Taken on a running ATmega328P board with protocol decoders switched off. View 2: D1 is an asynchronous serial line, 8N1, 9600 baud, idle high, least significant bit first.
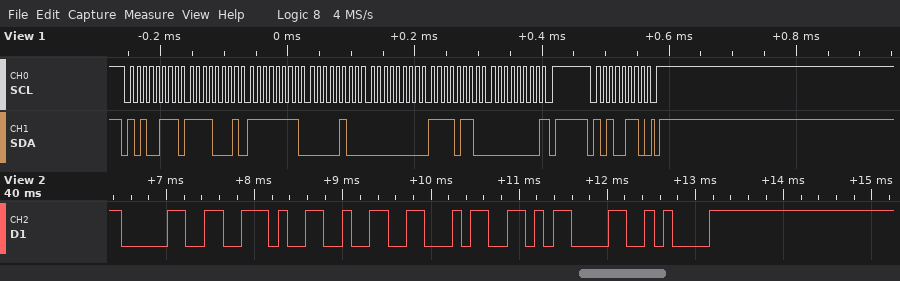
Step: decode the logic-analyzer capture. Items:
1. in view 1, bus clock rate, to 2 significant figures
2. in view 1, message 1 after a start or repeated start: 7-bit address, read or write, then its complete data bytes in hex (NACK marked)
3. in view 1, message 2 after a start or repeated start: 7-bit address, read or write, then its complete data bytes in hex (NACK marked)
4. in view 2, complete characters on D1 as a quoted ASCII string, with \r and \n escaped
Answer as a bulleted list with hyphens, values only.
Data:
- 100 kHz
- 0x53 read: F1 FF 04 00 F6 00 NACK
- 0x53 write
- "0.24\r\n"
